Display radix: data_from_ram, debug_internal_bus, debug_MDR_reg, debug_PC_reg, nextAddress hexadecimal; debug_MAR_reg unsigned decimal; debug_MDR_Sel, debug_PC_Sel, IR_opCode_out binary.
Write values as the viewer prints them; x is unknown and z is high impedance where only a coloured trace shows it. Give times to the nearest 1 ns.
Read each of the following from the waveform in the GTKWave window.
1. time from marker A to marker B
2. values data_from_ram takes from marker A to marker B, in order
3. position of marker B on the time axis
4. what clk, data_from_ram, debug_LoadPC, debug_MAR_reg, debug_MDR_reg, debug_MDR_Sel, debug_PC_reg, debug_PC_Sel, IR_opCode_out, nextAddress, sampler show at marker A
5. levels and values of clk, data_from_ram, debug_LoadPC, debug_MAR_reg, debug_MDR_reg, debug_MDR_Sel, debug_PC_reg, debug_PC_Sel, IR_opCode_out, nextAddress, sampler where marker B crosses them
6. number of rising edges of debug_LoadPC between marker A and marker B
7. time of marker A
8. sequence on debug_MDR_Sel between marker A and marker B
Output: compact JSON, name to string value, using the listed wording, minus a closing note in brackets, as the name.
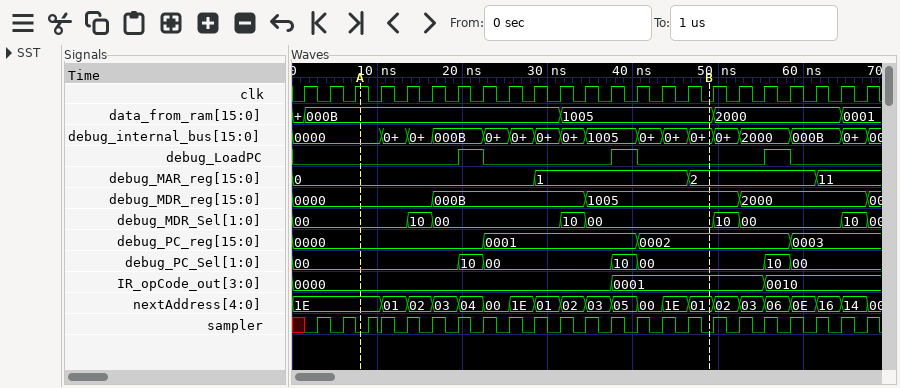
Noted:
{"time from marker A to marker B": "41 ns", "values data_from_ram takes from marker A to marker B, in order": "000B, 1005", "position of marker B on the time axis": "49 ns", "what clk, data_from_ram, debug_LoadPC, debug_MAR_reg, debug_MDR_reg, debug_MDR_Sel, debug_PC_reg, debug_PC_Sel, IR_opCode_out, nextAddress, sampler show at marker A": "clk=1, data_from_ram=000B, debug_LoadPC=0, debug_MAR_reg=0, debug_MDR_reg=0000, debug_MDR_Sel=00, debug_PC_reg=0000, debug_PC_Sel=00, IR_opCode_out=0000, nextAddress=1E, sampler=0", "levels and values of clk, data_from_ram, debug_LoadPC, debug_MAR_reg, debug_MDR_reg, debug_MDR_Sel, debug_PC_reg, debug_PC_Sel, IR_opCode_out, nextAddress, sampler where marker B crosses them": "clk=0, data_from_ram=1005, debug_LoadPC=0, debug_MAR_reg=2, debug_MDR_reg=1005, debug_MDR_Sel=00, debug_PC_reg=0002, debug_PC_Sel=00, IR_opCode_out=0001, nextAddress=01, sampler=0", "number of rising edges of debug_LoadPC between marker A and marker B": "2", "time of marker A": "8 ns", "sequence on debug_MDR_Sel between marker A and marker B": "00, 10, 00, 10, 00"}
